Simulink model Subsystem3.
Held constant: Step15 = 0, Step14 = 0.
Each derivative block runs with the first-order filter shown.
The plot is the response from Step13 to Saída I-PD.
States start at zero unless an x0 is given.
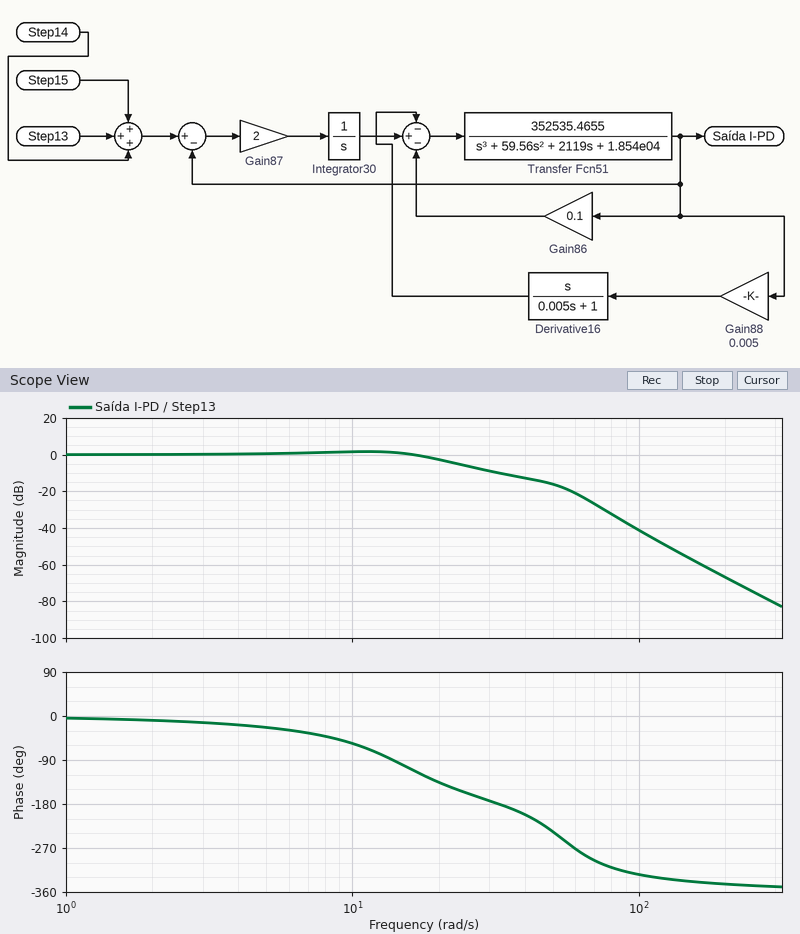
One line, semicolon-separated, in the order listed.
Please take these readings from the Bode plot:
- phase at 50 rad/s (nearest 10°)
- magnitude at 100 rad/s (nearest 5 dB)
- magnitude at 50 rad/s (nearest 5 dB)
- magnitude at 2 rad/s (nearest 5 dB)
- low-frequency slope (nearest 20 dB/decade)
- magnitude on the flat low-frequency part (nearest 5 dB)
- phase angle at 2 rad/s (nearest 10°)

-240°; -40 dB; -15 dB; 0 dB; 0 dB/decade; 0 dB; -10°
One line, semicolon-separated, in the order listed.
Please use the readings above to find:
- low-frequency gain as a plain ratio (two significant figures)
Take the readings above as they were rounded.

1.0
